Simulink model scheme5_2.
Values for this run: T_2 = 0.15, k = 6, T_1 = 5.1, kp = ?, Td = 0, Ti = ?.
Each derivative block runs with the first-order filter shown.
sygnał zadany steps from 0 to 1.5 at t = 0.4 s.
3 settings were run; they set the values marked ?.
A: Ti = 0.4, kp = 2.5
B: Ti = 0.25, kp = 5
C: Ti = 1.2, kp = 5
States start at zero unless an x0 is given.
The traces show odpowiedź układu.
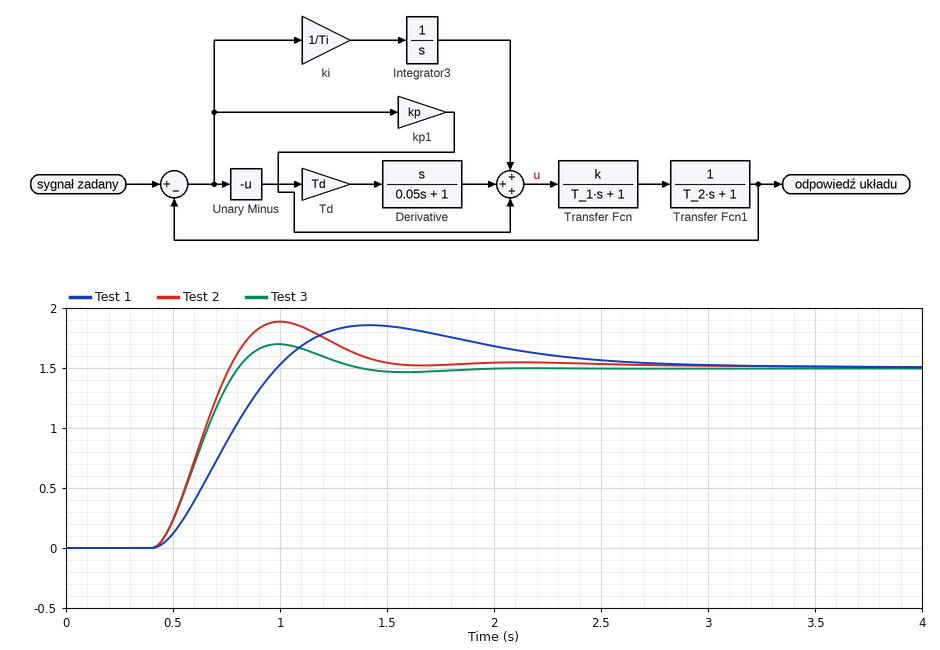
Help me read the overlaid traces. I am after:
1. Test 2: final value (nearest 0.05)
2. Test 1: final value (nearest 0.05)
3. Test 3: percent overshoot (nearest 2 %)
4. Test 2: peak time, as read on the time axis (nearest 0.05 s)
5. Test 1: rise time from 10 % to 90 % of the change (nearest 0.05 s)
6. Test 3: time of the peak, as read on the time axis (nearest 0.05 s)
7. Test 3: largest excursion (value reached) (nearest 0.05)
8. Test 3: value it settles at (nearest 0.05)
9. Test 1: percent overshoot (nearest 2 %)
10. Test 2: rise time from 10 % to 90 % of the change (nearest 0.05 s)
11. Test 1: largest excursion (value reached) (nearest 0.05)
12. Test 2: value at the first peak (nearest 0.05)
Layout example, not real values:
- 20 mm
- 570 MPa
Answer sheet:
- 1.50
- 1.50
- 14 %
- 1.00 s
- 0.40 s
- 1.00 s
- 1.70
- 1.50
- 24 %
- 0.25 s
- 1.85
- 1.90
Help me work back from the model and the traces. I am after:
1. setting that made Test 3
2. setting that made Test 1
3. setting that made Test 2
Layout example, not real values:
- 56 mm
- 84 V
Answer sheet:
- C
- A
- B
